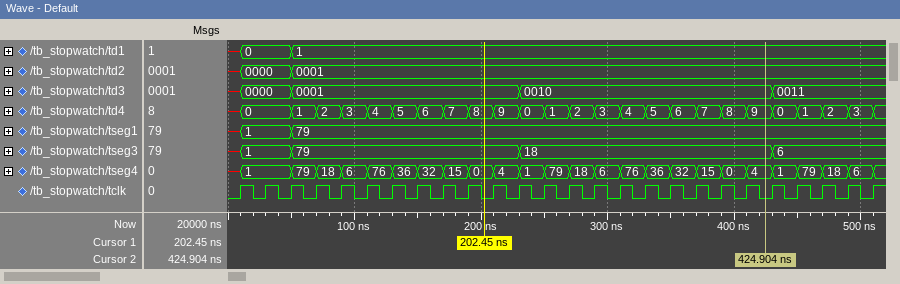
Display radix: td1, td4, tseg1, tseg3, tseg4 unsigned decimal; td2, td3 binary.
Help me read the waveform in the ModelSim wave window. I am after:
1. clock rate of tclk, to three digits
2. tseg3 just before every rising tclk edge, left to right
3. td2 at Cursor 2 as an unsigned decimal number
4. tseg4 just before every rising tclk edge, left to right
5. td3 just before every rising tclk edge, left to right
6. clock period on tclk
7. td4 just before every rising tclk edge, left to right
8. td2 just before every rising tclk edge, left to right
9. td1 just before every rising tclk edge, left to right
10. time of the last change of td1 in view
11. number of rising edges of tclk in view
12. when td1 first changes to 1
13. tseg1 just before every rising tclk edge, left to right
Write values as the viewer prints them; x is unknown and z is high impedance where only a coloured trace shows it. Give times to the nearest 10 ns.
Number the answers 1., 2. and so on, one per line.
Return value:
1. 50.0 MHz
2. x, 1, 1, 79, 79, 79, 79, 79, 79, 79, 79, 79, 18, 18, 18, 18, 18, 18, 18, 18, 18, 18, 6, 6, 6, 6
3. 1
4. x, 1, 1, 79, 18, 6, 76, 36, 32, 15, 0, 4, 1, 79, 18, 6, 76, 36, 32, 15, 0, 4, 1, 79, 18, 6
5. x, 0000, 0000, 0001, 0001, 0001, 0001, 0001, 0001, 0001, 0001, 0001, 0010, 0010, 0010, 0010, 0010, 0010, 0010, 0010, 0010, 0010, 0011, 0011, 0011, 0011
6. 20 ns
7. x, 0, 0, 1, 2, 3, 4, 5, 6, 7, 8, 9, 0, 1, 2, 3, 4, 5, 6, 7, 8, 9, 0, 1, 2, 3
8. x, 0000, 0000, 0001, 0001, 0001, 0001, 0001, 0001, 0001, 0001, 0001, 0001, 0001, 0001, 0001, 0001, 0001, 0001, 0001, 0001, 0001, 0001, 0001, 0001, 0001
9. x, 0, 0, 1, 1, 1, 1, 1, 1, 1, 1, 1, 1, 1, 1, 1, 1, 1, 1, 1, 1, 1, 1, 1, 1, 1
10. 50 ns
11. 26
12. 50 ns
13. x, 1, 1, 79, 79, 79, 79, 79, 79, 79, 79, 79, 79, 79, 79, 79, 79, 79, 79, 79, 79, 79, 79, 79, 79, 79
